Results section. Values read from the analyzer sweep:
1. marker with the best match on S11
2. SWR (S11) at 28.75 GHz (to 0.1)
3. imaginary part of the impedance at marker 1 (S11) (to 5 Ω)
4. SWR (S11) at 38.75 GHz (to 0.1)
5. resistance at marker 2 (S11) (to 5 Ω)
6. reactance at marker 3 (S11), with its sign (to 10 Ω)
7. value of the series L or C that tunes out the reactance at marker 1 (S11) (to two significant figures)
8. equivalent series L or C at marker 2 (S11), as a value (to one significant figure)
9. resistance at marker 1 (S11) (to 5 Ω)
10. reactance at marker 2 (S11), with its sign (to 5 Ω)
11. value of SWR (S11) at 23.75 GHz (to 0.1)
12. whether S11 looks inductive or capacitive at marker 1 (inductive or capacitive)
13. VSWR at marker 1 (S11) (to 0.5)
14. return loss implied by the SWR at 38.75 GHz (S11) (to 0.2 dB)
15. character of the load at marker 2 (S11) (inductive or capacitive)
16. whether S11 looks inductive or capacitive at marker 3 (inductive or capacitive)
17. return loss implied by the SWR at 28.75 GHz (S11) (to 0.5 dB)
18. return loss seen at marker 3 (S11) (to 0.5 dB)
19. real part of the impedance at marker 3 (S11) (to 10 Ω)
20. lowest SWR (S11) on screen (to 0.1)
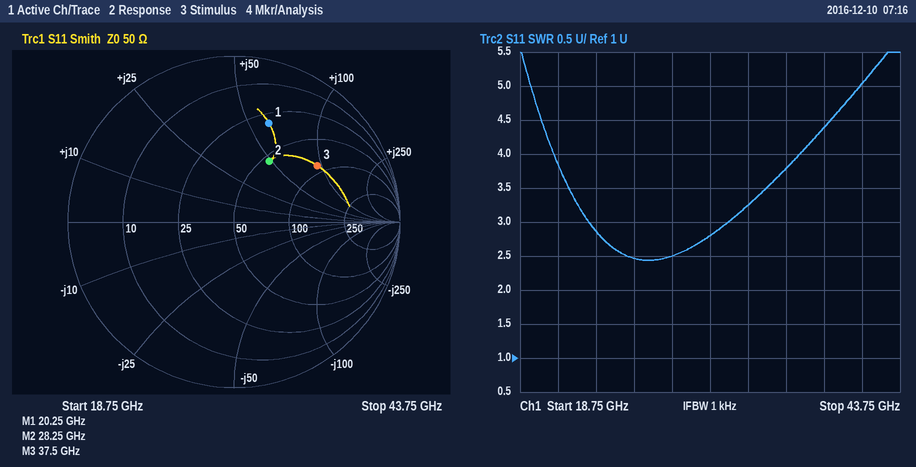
marker 2
2.5
+60 Ω
4.4
55 Ω
+90 Ω
130 fF
300 pH
30 Ω
+50 Ω
2.9
inductive
4.5
4.0 dB
inductive
inductive
7.5 dB
4.5 dB
90 Ω
2.4
